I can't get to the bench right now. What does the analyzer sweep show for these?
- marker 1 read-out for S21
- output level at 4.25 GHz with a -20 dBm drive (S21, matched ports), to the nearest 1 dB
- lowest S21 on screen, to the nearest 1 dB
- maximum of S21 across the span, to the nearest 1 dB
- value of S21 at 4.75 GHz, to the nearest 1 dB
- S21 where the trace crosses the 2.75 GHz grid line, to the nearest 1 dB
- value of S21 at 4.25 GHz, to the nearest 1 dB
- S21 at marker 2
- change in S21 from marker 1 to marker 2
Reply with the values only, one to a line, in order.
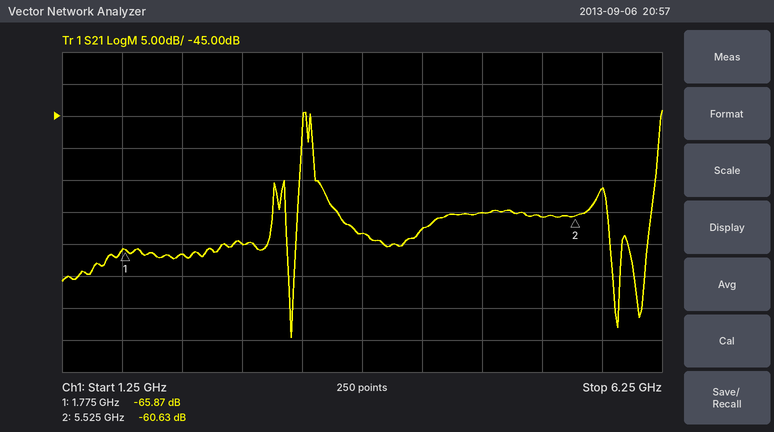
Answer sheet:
-65.87 dB
-83 dBm
-80 dB
-44 dB
-60 dB
-65 dB
-63 dB
-60.63 dB
5.24 dB
